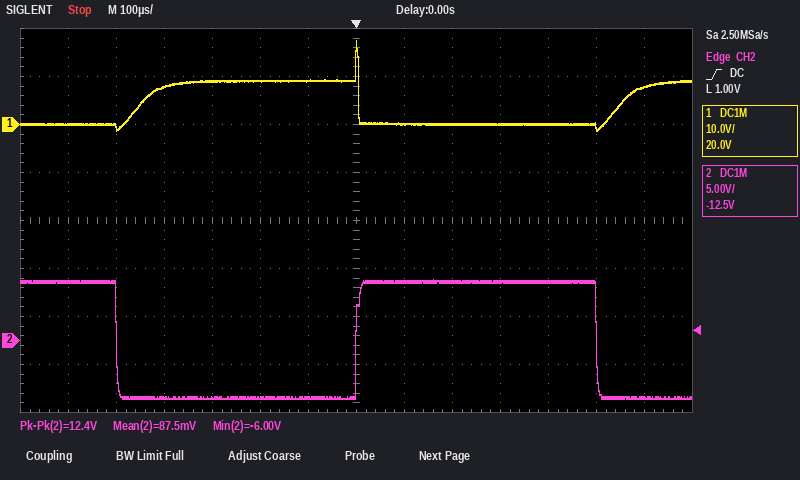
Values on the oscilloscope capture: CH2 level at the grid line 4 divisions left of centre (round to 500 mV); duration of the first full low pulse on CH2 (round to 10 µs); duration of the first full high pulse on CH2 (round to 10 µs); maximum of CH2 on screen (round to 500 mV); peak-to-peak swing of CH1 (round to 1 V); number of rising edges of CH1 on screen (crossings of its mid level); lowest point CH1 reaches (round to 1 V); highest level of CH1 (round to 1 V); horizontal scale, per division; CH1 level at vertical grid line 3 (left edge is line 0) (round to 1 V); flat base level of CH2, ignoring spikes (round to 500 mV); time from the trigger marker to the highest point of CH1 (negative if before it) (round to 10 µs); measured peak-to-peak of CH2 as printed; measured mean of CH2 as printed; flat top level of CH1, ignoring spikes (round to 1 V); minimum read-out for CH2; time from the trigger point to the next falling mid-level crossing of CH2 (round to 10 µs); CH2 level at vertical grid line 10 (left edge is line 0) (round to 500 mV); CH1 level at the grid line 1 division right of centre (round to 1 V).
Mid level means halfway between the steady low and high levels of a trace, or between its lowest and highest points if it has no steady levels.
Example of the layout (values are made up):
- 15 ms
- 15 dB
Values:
- -6.0 V
- 500 µs
- 500 µs
- 6.5 V
- 19 V
- 2
- -1 V
- 18 V
- 100 µs
- 8 V
- -6.0 V
- 0 µs
- 12.4 V
- 87.5 mV
- 9 V
- -6.00 V
- 500 µs
- 6.0 V
- 0 V
